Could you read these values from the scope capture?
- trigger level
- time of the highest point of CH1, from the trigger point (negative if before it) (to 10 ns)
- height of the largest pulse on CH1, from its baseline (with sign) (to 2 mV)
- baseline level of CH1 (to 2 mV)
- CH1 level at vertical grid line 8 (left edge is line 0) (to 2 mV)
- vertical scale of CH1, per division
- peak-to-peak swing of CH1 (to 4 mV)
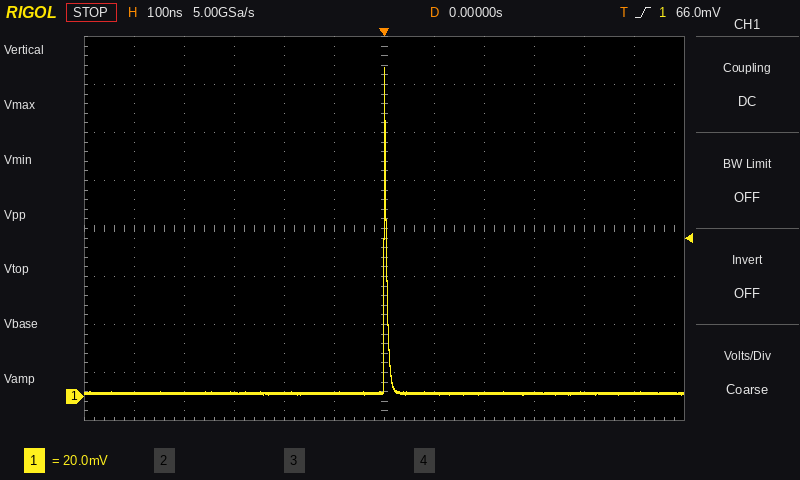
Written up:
66.0 mV
0 ns
+136 mV
2 mV
2 mV
20 mV
136 mV
